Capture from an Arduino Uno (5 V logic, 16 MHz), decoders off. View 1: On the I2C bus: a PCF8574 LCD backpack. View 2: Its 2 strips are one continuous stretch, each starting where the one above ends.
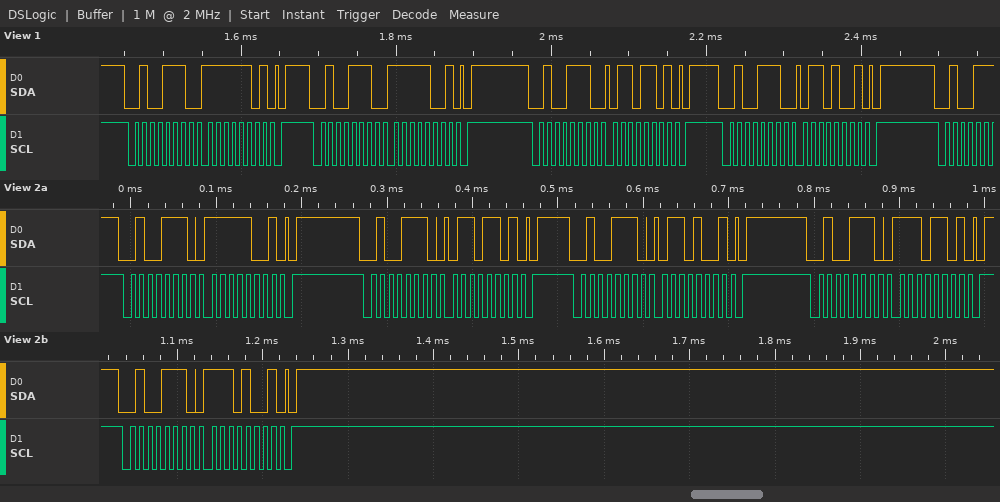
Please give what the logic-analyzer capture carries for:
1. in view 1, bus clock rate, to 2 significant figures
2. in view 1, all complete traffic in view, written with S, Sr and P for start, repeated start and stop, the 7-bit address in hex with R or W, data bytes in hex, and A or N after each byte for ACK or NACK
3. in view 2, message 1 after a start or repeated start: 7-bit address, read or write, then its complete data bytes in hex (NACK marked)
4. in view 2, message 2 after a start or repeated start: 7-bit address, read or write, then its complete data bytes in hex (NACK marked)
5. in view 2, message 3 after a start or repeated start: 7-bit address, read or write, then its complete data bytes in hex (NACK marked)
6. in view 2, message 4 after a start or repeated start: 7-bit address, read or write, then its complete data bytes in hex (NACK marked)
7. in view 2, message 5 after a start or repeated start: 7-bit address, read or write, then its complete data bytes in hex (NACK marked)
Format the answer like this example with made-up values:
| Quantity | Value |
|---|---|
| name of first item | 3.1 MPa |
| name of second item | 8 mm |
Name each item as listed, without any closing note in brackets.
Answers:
| Quantity | Value |
|---|---|
| in view 1, bus clock rate, to 2 significant figures | 100 kHz |
| in view 1, all complete traffic in view, written with S, Sr and P for start, repeated start and stop, the 7-bit address in hex with R or W, data bytes in hex, and A or N after each byte for ACK or NACK | S 27W A FD A P S 27W A F9 A P S 27W A 6D A P S 27W A 69 A P |
| in view 2, message 1 after a start or repeated start: 7-bit address, read or write, then its complete data bytes in hex | 0x27 write: F9 |
| in view 2, message 2 after a start or repeated start: 7-bit address, read or write, then its complete data bytes in hex | 0x27 write: 6D |
| in view 2, message 3 after a start or repeated start: 7-bit address, read or write, then its complete data bytes in hex | 0x27 write: 69 |
| in view 2, message 4 after a start or repeated start: 7-bit address, read or write, then its complete data bytes in hex | 0x27 write: ED |
| in view 2, message 5 after a start or repeated start: 7-bit address, read or write, then its complete data bytes in hex | 0x27 write: E9 |
